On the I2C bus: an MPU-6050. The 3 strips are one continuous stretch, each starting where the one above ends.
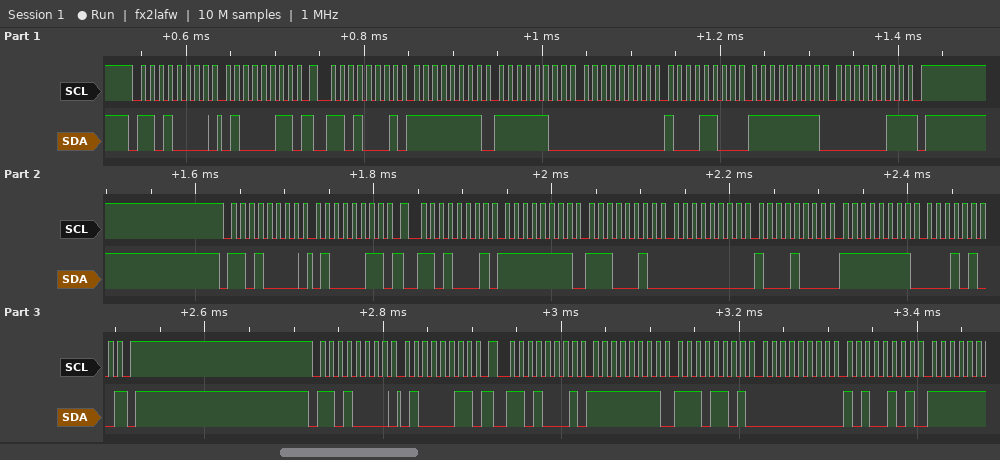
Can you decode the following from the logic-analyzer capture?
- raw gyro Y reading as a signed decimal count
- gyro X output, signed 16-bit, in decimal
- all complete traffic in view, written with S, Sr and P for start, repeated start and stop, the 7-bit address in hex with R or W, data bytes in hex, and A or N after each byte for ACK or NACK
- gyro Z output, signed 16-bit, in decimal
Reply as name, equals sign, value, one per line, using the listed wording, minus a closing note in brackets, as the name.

raw gyro Y reading as a signed decimal count = 140
gyro X output, signed 16-bit, in decimal = -4
all complete traffic in view, written with S, Sr and P for start, repeated start and stop, the 7-bit address in hex with R or W, data bytes in hex, and A or N after each byte for ACK or NACK = S 68W A 43 A Sr 68R A FF A FC A 00 A 8C A FF A 03 N P S 68W A 43 A Sr 68R A FF A E2 A 00 A 88 A FF A 14 N P S 68W A 43 A Sr 68R A FF A ED A 00 A A5 A
gyro Z output, signed 16-bit, in decimal = -253
